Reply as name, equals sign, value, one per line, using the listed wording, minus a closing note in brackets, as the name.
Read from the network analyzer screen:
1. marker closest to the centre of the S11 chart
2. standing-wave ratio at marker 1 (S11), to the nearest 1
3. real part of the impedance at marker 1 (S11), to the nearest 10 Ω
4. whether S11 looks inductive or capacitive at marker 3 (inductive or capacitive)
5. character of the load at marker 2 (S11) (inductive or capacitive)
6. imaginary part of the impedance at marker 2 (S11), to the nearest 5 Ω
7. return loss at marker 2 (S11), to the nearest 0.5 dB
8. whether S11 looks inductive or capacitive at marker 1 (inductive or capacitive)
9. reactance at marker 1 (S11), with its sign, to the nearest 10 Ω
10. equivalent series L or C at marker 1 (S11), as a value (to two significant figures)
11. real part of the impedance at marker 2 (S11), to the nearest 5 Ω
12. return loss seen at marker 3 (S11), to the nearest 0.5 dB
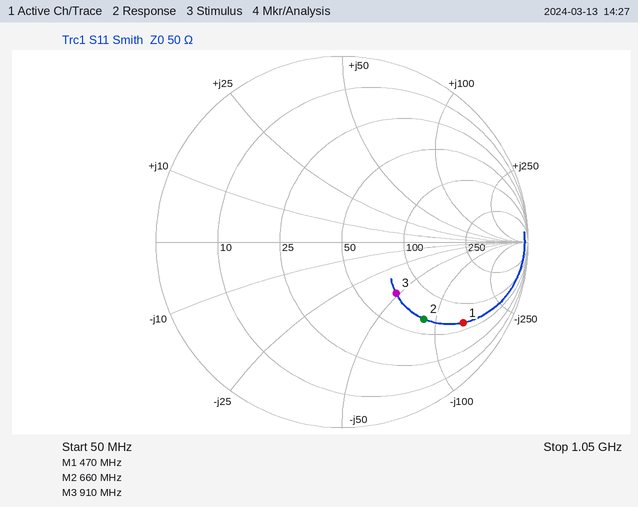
marker closest to the centre of the S11 chart = marker 3
standing-wave ratio at marker 1 (S11), to the nearest 1 = 8
real part of the impedance at marker 1 (S11), to the nearest 10 Ω = 60 Ω
whether S11 looks inductive or capacitive at marker 3 = capacitive
character of the load at marker 2 (S11) = capacitive
imaginary part of the impedance at marker 2 (S11), to the nearest 5 Ω = -85 Ω
return loss at marker 2 (S11), to the nearest 0.5 dB = 4.5 dB
whether S11 looks inductive or capacitive at marker 1 = capacitive
reactance at marker 1 (S11), with its sign, to the nearest 10 Ω = -140 Ω
equivalent series L or C at marker 1 (S11), as a value = 2.4 pF
real part of the impedance at marker 2 (S11), to the nearest 5 Ω = 65 Ω
return loss seen at marker 3 (S11), to the nearest 0.5 dB = 8.0 dB
